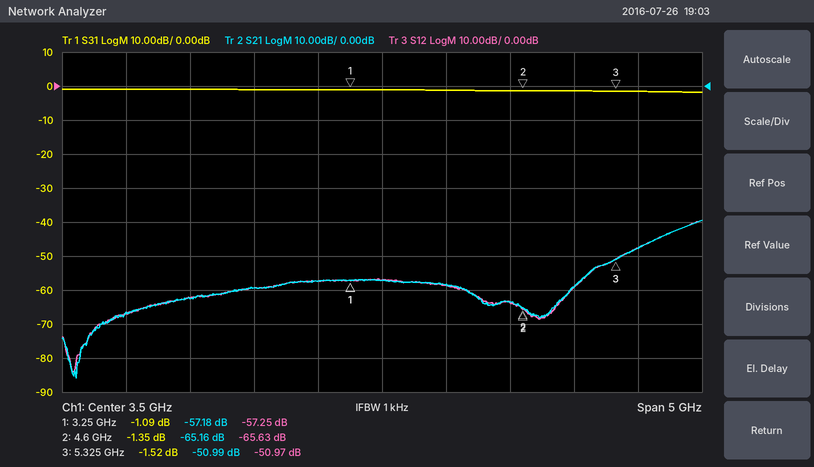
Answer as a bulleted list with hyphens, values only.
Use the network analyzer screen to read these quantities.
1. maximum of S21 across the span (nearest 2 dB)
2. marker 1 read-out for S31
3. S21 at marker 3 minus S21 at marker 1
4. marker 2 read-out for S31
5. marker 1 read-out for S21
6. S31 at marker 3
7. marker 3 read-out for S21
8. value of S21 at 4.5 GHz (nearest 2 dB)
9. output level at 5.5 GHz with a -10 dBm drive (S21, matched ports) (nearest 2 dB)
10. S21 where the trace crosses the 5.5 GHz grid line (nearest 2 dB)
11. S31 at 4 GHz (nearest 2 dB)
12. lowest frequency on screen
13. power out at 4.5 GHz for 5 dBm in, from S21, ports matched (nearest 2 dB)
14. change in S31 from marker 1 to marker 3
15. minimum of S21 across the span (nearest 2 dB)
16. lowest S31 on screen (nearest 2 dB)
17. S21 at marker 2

- -40 dB
- -1.09 dB
- 6.19 dB
- -1.35 dB
- -57.18 dB
- -1.52 dB
- -50.99 dB
- -64 dB
- -58 dBm
- -48 dB
- -2 dB
- 1 GHz
- -58 dBm
- -0.43 dB
- -86 dB
- -2 dB
- -65.16 dB
